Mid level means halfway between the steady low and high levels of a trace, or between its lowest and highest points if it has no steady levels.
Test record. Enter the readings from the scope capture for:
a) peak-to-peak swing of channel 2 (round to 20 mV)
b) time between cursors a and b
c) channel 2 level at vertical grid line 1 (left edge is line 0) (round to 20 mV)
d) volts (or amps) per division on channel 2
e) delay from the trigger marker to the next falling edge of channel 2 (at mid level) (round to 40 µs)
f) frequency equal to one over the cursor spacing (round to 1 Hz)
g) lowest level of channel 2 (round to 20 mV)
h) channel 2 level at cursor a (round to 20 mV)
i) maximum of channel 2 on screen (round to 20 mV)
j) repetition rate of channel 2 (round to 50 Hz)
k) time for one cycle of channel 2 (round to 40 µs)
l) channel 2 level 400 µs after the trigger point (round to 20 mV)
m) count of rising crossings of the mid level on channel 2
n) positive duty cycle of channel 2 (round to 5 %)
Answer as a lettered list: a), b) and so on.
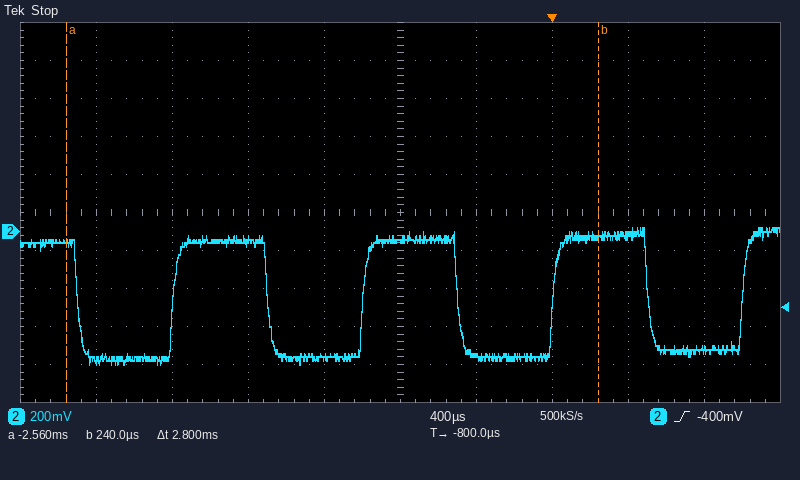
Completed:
a) 720 mV
b) 2.8 ms
c) -680 mV
d) 200 mV
e) 520 µs
f) 357 Hz
g) -700 mV
h) -60 mV
i) 20 mV
j) 1.00 kHz
k) 1.00 ms
l) -20 mV
m) 4
n) 50 %
